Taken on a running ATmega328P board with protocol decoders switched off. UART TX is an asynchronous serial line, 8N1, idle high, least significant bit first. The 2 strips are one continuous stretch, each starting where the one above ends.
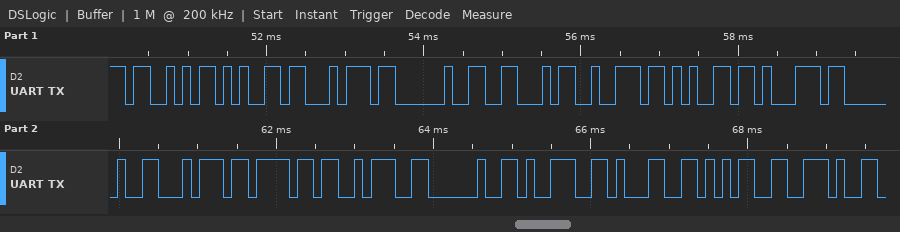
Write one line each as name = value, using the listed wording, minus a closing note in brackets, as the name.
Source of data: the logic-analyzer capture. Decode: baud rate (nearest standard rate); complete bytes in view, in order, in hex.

baud rate = 9600 baud
complete bytes in view, in order, in hex = 0x53 0x65 0x74 0x20 0x46 0x72 0x65 0x71 0x20 0x74 0x6F 0x3A 0x20 0x39 0x31 0x35 0x2E
